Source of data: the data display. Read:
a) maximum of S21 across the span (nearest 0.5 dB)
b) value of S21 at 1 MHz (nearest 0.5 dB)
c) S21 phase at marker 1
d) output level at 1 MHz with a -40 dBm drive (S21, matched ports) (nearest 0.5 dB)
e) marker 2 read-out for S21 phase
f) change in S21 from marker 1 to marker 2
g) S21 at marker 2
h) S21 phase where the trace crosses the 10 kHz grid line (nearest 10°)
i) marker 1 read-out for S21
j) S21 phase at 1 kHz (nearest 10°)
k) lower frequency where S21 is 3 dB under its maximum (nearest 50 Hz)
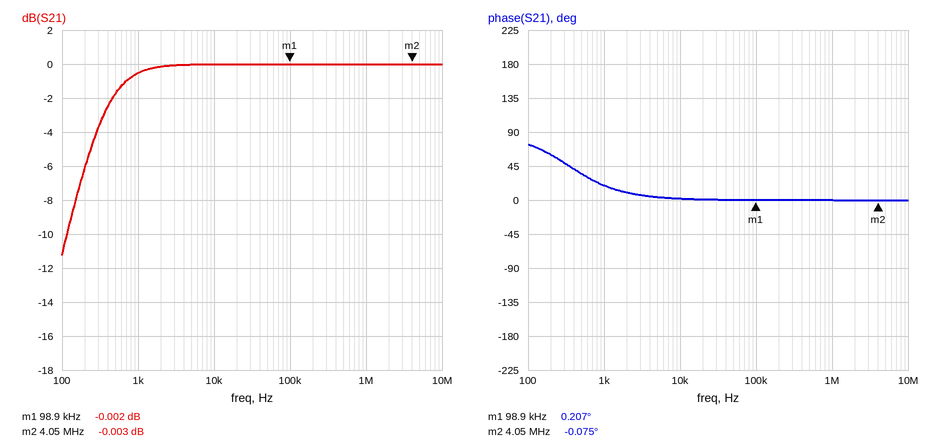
0.0 dB
0.0 dB
0.207°
-40.0 dBm
-0.075°
-0.001 dB
-0.003 dB
0°
-0.002 dB
20°
350 Hz
